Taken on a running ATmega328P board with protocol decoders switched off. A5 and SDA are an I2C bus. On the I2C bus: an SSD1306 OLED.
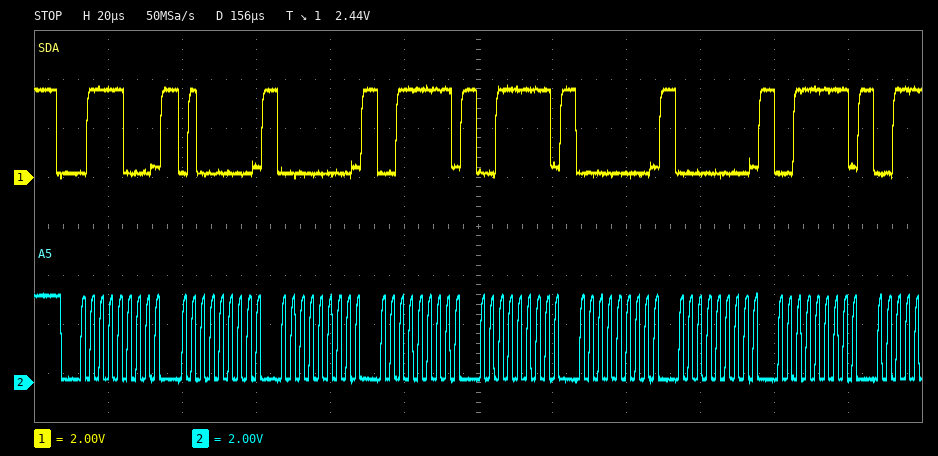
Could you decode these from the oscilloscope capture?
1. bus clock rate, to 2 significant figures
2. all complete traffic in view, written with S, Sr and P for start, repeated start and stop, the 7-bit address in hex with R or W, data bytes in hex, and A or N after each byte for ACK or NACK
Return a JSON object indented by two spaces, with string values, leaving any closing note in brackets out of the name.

{
  "bus clock rate, to 2 significant figures": "400 kHz",
  "all complete traffic in view, written with S, Sr and P for start, repeated start and stop, the 7-bit address in hex with R or W, data bytes in hex, and A or N after each byte for ACK or NACK": "S 3CW A 40 A 00 A 3F A 3F A 00 A 00 A 3F A"
}
